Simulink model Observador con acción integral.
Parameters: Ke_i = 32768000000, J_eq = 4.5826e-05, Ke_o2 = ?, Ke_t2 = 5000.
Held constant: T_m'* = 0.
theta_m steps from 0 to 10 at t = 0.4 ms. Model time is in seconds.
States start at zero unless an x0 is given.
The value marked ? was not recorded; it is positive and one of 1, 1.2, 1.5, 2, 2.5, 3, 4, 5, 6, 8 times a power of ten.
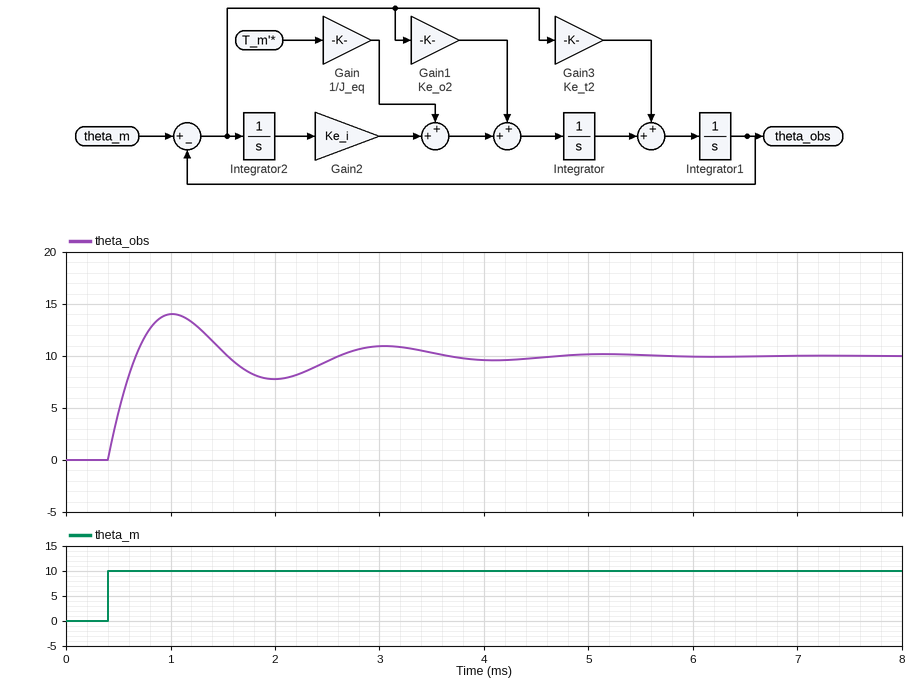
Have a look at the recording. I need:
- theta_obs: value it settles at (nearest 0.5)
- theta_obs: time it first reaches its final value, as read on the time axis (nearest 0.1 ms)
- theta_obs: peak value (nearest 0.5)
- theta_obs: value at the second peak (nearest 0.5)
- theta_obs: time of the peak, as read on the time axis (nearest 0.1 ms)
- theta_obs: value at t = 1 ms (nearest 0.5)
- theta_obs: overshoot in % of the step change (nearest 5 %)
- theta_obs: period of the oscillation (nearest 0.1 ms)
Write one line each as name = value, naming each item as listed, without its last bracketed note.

theta_obs: value it settles at = 10.0
theta_obs: time it first reaches its final value, as read on the time axis = 0.7 ms
theta_obs: peak value = 14.0
theta_obs: value at the second peak = 11.0
theta_obs: time of the peak, as read on the time axis = 1.0 ms
theta_obs: value at t = 1 ms = 14.0
theta_obs: overshoot in % of the step change = 40 %
theta_obs: period of the oscillation = 2.0 ms
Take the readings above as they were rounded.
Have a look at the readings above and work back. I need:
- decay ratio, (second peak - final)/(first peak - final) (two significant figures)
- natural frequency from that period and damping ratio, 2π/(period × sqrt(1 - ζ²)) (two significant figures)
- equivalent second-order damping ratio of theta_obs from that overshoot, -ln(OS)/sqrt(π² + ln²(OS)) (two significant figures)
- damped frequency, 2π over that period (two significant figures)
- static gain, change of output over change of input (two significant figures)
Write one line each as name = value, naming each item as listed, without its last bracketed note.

decay ratio, (second peak - final)/(first peak - final) = 0.25
natural frequency from that period and damping ratio, 2π/(period × sqrt(1 - ζ²)) = 3.3 rad/ms
equivalent second-order damping ratio of theta_obs from that overshoot, -ln(OS)/sqrt(π² + ln²(OS)) = 0.28
damped frequency, 2π over that period = 3.1 rad/ms
static gain, change of output over change of input = 1.0
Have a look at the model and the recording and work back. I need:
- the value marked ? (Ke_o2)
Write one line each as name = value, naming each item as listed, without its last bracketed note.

the value marked ? = 1.5e+07
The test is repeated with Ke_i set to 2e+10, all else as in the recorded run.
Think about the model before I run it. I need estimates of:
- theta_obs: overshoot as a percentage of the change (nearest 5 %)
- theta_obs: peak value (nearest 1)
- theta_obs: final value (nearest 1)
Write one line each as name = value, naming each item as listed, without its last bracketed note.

theta_obs: overshoot as a percentage of the change = 35 %
theta_obs: peak value = 13
theta_obs: final value = 10
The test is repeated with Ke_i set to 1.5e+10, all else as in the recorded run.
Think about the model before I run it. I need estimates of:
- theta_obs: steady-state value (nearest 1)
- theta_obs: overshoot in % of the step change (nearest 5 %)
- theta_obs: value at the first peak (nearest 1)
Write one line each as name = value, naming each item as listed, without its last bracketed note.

theta_obs: steady-state value = 10
theta_obs: overshoot in % of the step change = 30 %
theta_obs: value at the first peak = 13
